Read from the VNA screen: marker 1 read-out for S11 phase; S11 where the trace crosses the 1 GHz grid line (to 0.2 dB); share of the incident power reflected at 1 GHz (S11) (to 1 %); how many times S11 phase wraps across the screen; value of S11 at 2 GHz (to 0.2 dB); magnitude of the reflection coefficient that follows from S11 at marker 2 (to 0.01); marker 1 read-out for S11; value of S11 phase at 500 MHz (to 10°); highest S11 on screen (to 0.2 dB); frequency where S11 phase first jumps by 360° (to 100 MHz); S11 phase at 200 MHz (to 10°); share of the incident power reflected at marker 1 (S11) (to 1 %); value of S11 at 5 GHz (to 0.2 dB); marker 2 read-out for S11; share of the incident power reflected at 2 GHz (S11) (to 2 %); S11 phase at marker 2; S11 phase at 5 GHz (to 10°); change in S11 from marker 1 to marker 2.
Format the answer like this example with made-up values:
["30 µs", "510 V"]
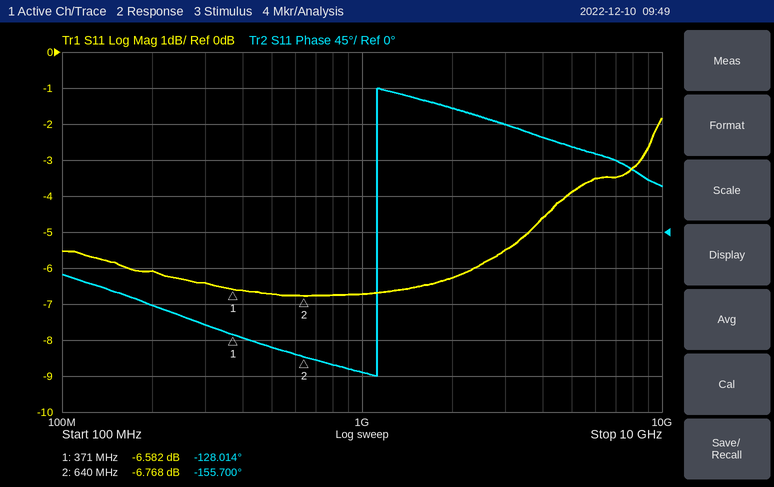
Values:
["-128.014°", "-6.8 dB", "21 %", "1", "-6.2 dB", "0.46", "-6.582 dB", "-140°", "-1.8 dB", "1.1 GHz", "-90°", "22 %", "-3.8 dB", "-6.768 dB", "24 %", "-155.700°", "110°", "-0.186 dB"]
